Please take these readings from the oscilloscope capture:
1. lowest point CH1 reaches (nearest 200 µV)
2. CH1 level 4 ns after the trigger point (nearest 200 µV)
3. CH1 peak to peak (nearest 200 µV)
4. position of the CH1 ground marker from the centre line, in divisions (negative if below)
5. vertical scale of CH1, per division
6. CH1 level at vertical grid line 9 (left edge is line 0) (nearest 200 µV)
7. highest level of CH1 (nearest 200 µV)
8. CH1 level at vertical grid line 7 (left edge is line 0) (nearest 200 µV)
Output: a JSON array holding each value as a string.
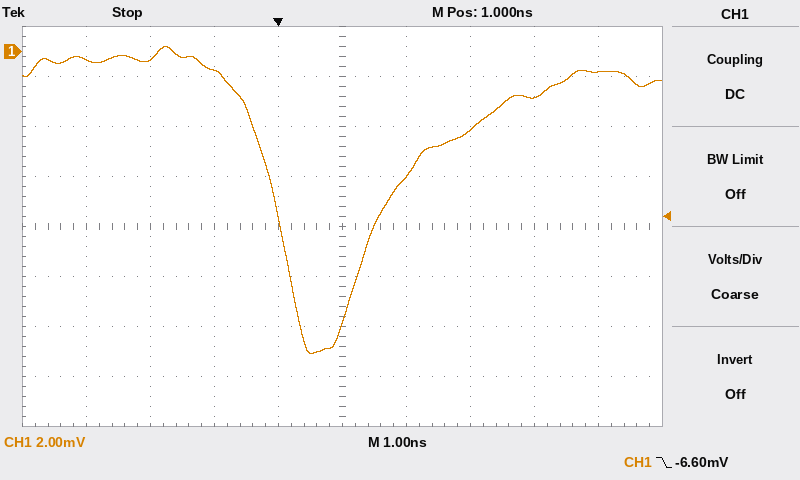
["-12.0 mV", "-1.8 mV", "12.2 mV", "+3.5 div", "2 mV", "-800 µV", "200 µV", "-3.2 mV"]
